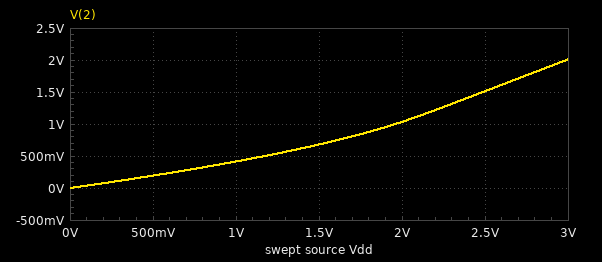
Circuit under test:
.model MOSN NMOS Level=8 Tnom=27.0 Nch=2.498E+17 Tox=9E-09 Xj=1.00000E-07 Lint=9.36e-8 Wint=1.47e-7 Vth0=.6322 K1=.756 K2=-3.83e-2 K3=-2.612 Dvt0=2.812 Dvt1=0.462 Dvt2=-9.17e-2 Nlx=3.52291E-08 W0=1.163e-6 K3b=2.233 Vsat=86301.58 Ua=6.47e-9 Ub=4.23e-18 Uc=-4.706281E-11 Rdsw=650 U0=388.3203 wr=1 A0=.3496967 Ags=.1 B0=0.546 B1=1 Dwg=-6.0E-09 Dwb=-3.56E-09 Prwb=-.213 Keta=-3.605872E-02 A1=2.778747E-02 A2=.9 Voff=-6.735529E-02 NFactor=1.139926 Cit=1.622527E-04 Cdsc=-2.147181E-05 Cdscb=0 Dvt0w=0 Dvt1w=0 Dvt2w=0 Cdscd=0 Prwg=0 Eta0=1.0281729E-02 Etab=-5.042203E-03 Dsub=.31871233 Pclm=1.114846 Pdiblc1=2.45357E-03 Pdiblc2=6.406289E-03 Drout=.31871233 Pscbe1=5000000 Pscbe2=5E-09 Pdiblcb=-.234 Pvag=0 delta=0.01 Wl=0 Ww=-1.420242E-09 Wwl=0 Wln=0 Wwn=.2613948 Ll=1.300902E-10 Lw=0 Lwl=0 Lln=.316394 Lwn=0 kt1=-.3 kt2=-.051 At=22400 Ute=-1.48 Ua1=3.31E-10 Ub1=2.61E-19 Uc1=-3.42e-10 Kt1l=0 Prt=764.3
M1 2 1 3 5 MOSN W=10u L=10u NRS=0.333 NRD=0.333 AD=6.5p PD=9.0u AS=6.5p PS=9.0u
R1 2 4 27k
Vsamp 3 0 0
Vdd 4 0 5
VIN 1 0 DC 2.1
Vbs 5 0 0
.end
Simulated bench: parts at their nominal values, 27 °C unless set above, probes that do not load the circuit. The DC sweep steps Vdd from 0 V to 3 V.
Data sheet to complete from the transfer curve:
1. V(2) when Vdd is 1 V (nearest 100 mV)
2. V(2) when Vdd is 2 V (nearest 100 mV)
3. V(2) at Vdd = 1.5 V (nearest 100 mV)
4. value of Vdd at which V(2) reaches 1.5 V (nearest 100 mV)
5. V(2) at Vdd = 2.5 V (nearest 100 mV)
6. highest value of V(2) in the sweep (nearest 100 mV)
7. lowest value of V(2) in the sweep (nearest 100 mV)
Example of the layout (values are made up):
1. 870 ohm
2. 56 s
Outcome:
1. 400 mV
2. 1.0 V
3. 700 mV
4. 2.5 V
5. 1.5 V
6. 2.0 V
7. 0 V
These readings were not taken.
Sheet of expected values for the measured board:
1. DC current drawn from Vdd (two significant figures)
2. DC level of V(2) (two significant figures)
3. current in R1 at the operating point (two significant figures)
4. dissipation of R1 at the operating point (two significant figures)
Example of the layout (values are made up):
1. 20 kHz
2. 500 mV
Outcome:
1. 37 µA
2. 4.0 V
3. 37 µA
4. 37 µW
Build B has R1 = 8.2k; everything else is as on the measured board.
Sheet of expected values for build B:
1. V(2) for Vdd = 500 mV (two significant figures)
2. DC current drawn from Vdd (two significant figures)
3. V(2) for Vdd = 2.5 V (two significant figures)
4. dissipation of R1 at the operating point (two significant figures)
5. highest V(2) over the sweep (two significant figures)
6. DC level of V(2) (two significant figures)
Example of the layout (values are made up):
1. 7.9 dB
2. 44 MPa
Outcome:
1. 350 mV
2. 37 µA
3. 2.2 V
4. 11 µW
5. 2.7 V
6. 4.7 V
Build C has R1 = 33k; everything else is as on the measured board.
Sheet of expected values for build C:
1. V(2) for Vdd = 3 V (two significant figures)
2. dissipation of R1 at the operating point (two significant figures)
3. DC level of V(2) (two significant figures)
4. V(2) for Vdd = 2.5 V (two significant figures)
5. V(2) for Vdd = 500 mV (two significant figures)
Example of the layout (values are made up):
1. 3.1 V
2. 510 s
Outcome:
1. 1.8 V
2. 45 µW
3. 3.8 V
4. 1.3 V
5. 170 mV
